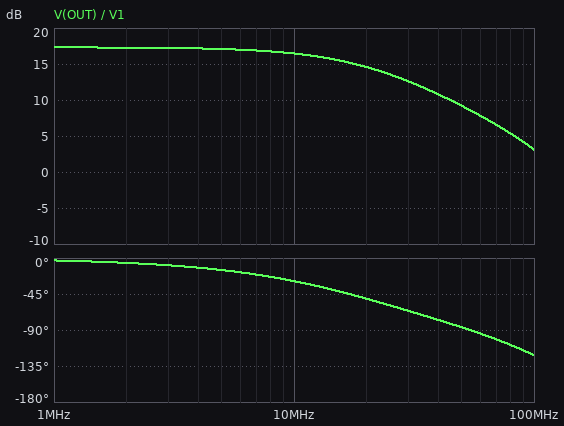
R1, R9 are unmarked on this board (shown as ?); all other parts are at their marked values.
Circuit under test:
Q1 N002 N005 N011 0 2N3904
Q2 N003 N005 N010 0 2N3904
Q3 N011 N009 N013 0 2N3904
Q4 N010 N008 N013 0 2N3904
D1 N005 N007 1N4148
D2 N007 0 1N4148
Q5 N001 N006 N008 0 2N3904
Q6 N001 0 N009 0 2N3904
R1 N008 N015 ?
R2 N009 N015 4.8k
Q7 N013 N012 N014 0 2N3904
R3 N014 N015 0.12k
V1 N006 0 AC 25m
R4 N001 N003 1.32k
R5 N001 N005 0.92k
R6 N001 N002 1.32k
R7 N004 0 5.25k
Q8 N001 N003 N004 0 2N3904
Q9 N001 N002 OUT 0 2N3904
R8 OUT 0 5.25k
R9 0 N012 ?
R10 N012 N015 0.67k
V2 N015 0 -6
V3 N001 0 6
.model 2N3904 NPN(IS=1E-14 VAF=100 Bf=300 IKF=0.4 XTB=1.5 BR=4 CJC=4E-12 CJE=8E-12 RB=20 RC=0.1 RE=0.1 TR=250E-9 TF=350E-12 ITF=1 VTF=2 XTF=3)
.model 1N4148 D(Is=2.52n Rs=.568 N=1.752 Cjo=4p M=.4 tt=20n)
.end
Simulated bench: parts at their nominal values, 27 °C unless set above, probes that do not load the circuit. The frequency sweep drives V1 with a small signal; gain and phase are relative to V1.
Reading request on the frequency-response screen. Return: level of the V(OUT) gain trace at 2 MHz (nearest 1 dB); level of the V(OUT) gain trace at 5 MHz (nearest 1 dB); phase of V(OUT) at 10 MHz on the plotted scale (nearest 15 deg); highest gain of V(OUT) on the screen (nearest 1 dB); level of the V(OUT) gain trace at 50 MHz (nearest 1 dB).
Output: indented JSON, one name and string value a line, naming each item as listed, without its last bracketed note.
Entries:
{
  "level of the V(OUT) gain trace at 2 MHz": "17 dB",
  "level of the V(OUT) gain trace at 5 MHz": "17 dB",
  "phase of V(OUT) at 10 MHz on the plotted scale": "-30 deg",
  "highest gain of V(OUT) on the screen": "17 dB",
  "level of the V(OUT) gain trace at 50 MHz": "9 dB"
}
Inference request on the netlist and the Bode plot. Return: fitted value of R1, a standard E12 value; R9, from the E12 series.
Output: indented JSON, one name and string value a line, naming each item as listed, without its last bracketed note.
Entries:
{
  "fitted value of R1, a standard E12 value": "1.5 kΩ",
  "R9, from the E12 series": "4.7 kΩ"
}
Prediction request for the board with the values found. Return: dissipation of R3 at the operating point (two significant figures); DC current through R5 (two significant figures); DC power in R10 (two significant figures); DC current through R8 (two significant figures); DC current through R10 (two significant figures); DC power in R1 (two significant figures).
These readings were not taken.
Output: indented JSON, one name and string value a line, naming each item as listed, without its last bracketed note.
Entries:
{
  "dissipation of R3 at the operating point": "80 µW",
  "DC current through R5": "5.1 mA",
  "DC power in R10": "830 µW",
  "DC current through R8": "860 µA",
  "DC current through R10": "1.1 mA",
  "DC power in R1": "19 mW"
}
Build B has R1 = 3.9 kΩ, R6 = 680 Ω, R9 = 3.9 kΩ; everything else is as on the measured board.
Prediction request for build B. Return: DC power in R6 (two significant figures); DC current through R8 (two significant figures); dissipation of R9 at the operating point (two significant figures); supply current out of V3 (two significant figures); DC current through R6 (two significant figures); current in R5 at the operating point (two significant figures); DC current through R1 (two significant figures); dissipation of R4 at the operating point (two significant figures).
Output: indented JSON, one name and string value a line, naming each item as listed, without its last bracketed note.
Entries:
{
  "DC power in R6": "610 µW",
  "DC current through R8": "900 µA",
  "dissipation of R9 at the operating point": "6.7 mW",
  "supply current out of V3": "11 mA",
  "DC current through R6": "950 µA",
  "current in R5 at the operating point": "5.1 mA",
  "DC current through R1": "1.4 mA",
  "dissipation of R4 at the operating point": "790 µW"
}
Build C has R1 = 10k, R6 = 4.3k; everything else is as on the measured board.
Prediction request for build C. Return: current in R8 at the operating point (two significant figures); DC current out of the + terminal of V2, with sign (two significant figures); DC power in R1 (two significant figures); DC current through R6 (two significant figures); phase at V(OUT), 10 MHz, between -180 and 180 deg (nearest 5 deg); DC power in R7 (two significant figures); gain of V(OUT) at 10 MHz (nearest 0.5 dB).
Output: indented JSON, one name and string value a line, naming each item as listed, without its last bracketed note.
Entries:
{
  "current in R8 at the operating point": "800 µA",
  "DC current out of the + terminal of V2, with sign": "-3.6 mA",
  "DC power in R1": "2.9 mW",
  "DC current through R6": "270 µA",
  "phase at V(OUT), 10 MHz, between -180 and 180 deg": "-70 deg",
  "DC power in R7": "4.1 mW",
  "gain of V(OUT) at 10 MHz": "24.0 dB"
}
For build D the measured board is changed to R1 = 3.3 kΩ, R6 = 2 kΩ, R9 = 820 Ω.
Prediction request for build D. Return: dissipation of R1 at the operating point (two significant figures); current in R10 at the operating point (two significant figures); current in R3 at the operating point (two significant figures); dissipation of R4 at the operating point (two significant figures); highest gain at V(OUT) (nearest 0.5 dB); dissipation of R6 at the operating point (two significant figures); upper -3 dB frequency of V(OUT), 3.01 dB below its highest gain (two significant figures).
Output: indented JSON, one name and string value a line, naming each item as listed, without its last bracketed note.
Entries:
{
  "dissipation of R1 at the operating point": "8.6 mW",
  "current in R10 at the operating point": "4.0 mA",
  "current in R3 at the operating point": "16 mA",
  "dissipation of R4 at the operating point": "39 mW",
  "highest gain at V(OUT)": "-7.0 dB",
  "dissipation of R6 at the operating point": "26 mW",
  "upper -3 dB frequency of V(OUT), 3.01 dB below its highest gain": "780 MHz"
}
